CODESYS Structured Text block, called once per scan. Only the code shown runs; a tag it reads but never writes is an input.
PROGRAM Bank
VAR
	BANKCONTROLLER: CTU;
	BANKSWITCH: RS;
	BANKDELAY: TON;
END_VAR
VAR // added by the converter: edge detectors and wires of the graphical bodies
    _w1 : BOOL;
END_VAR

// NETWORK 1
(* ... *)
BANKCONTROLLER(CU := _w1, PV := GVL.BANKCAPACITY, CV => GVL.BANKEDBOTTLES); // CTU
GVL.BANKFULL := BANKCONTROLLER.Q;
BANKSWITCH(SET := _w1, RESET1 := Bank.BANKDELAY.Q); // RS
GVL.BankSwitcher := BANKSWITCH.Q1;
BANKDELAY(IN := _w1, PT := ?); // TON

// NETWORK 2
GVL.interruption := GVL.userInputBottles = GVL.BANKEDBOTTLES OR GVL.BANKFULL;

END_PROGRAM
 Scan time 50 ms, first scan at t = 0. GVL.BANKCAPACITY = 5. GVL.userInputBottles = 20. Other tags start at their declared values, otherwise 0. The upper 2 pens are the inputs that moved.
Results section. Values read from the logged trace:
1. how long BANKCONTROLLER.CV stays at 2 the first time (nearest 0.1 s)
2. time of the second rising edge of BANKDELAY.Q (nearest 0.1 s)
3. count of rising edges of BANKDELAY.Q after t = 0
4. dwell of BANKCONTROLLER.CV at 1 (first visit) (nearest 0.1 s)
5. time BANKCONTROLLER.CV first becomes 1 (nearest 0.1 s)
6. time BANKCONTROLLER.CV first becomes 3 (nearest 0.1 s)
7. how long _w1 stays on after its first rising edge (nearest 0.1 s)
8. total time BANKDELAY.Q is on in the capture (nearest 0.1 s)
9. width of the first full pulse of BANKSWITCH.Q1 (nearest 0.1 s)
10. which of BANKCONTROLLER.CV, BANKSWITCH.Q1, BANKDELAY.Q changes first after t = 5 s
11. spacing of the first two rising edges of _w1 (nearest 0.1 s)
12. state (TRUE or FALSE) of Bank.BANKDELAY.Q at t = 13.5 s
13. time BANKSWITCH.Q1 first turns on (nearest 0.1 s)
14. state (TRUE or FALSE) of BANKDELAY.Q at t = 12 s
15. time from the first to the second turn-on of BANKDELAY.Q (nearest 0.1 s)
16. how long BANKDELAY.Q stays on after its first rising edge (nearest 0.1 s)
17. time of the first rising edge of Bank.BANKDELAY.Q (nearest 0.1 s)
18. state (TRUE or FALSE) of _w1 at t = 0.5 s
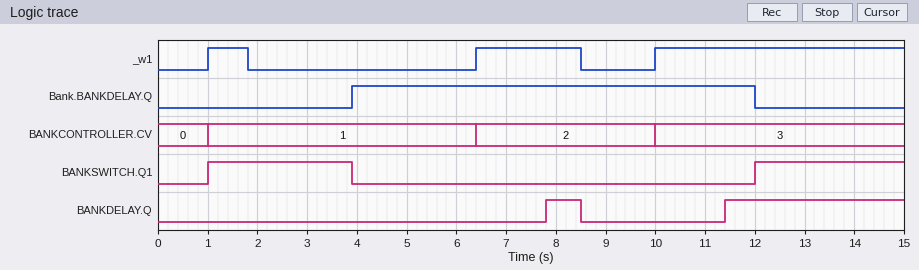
3.6 s
11.4 s
2
5.4 s
1.0 s
10.0 s
0.8 s
4.3 s
2.9 s
BANKCONTROLLER.CV
5.4 s
FALSE
1.0 s
TRUE
3.6 s
0.7 s
3.9 s
FALSE
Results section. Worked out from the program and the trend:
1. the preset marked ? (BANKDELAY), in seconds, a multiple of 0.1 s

1.4 s
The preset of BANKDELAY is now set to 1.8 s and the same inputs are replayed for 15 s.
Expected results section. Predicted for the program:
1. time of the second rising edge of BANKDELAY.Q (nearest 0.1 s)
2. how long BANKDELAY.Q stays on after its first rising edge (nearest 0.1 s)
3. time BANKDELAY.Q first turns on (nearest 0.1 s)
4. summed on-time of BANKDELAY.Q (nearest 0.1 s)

11.8 s
0.3 s
8.2 s
3.5 s
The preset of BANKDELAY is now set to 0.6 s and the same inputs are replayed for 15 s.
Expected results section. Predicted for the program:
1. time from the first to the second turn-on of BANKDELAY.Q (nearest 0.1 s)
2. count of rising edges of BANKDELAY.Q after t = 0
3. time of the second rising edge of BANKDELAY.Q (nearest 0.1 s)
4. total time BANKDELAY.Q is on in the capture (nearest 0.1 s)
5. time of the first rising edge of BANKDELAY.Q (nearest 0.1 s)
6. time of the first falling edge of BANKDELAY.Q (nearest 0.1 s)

5.4 s
3
7.0 s
6.1 s
1.6 s
1.8 s
